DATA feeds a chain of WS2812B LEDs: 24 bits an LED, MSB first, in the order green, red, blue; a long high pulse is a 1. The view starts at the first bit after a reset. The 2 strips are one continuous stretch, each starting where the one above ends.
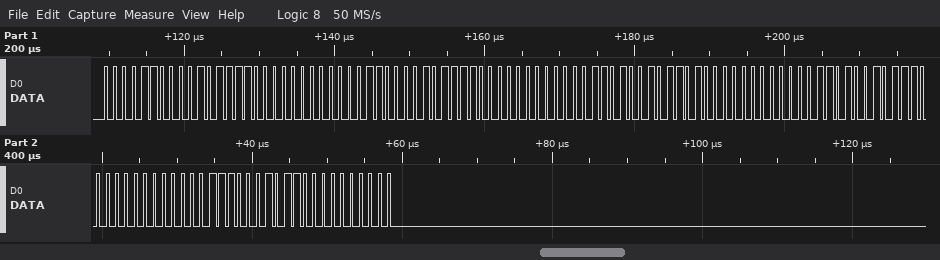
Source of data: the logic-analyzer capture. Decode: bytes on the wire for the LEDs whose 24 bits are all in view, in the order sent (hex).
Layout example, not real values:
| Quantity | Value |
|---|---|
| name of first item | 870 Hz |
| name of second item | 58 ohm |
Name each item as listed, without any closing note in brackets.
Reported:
| Quantity | Value |
|---|---|
| bytes on the wire for the LEDs whose 24 bits are all in view, in the order sent | 0C 2F 00 0C 2F 00 0D 2D 00 0D 2E 00 0E 2C 00 |
